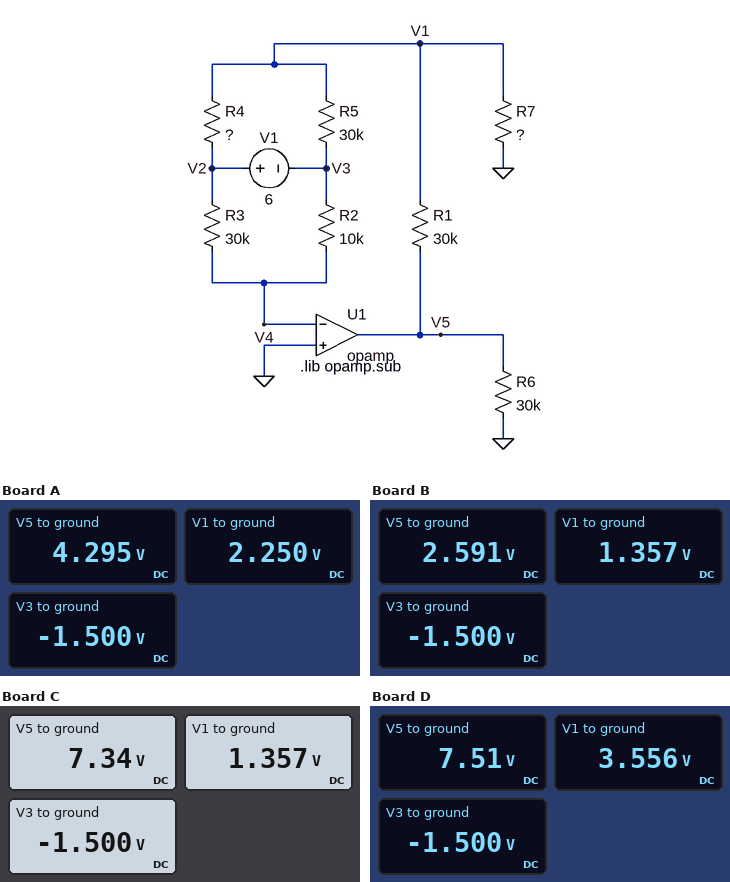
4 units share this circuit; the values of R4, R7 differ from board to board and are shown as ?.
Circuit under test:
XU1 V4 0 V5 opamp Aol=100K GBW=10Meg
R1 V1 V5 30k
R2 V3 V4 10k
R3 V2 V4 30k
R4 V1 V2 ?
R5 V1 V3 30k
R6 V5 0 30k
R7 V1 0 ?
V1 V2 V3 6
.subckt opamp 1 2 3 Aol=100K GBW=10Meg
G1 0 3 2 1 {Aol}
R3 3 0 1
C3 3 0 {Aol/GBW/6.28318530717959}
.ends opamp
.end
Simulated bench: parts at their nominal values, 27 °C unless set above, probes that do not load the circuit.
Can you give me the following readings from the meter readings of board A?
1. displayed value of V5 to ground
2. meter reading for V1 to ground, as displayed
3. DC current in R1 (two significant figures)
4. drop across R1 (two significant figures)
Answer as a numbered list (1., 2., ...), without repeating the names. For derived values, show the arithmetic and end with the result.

1. 4.295 V
2. 2.250 V
3. (4.295 V - 2.25 V) / 30 kΩ = 68 µA
4. 4.295 V - 2.25 V = 2.0 V
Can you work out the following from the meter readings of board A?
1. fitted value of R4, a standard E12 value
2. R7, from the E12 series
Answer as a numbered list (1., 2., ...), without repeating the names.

1. 18 kΩ
2. 33 kΩ
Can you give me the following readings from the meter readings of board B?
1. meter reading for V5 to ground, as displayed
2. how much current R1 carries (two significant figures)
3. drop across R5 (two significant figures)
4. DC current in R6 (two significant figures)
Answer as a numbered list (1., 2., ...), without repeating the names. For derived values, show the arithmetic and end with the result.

1. 2.591 V
2. (2.591 V - 1.357 V) / 30 kΩ = 41 µA
3. 1.357 V - (-1.5 V) = 2.9 V
4. (2.591 V) / 30 kΩ = 86 µA
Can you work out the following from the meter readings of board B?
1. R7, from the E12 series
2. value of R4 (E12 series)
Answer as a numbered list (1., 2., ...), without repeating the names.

1. 33 kΩ
2. 33 kΩ
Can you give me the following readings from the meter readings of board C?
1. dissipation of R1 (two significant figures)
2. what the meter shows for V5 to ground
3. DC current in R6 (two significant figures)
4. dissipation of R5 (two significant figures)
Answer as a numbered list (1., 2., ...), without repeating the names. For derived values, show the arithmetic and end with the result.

1. (7.34 V - 1.357 V)^2 / 30 kΩ = 1.2 mW
2. 7.34 V
3. (7.34 V) / 30 kΩ = 240 µA
4. (1.357 V - (-1.5 V))^2 / 30 kΩ = 270 µW
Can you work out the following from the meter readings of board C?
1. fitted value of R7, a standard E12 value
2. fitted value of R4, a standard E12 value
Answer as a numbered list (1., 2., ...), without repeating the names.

1. 6.8 kΩ
2. 33 kΩ
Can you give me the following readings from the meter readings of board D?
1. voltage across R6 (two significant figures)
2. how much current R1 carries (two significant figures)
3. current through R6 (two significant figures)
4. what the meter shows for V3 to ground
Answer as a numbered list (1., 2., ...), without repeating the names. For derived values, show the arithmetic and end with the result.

1. 7.51 V = 7.5 V
2. (7.51 V - 3.556 V) / 30 kΩ = 130 µA
3. (7.51 V) / 30 kΩ = 250 µA
4. -1.500 V
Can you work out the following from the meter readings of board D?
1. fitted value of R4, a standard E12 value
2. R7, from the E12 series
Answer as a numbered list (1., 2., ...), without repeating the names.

1. 5.6 kΩ
2. 27 kΩ
